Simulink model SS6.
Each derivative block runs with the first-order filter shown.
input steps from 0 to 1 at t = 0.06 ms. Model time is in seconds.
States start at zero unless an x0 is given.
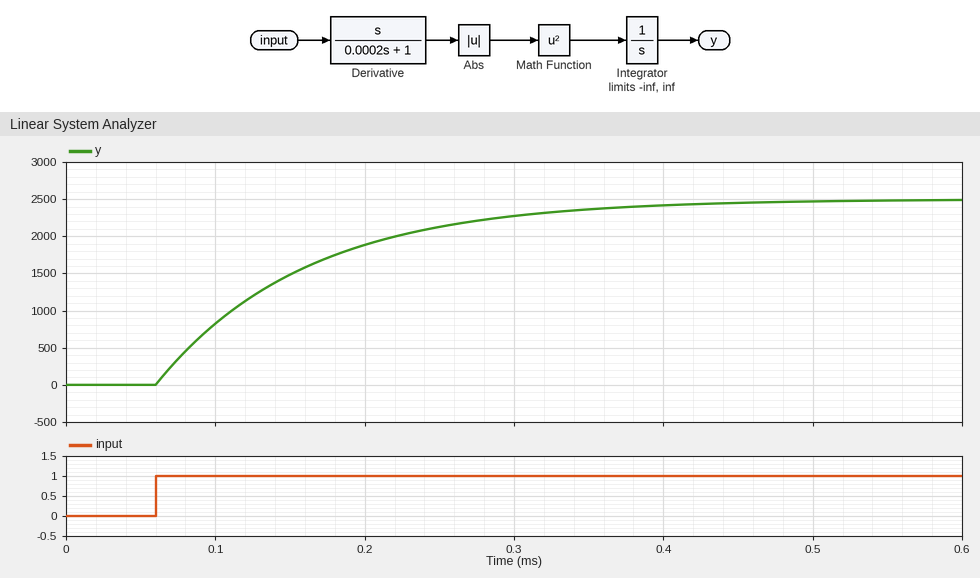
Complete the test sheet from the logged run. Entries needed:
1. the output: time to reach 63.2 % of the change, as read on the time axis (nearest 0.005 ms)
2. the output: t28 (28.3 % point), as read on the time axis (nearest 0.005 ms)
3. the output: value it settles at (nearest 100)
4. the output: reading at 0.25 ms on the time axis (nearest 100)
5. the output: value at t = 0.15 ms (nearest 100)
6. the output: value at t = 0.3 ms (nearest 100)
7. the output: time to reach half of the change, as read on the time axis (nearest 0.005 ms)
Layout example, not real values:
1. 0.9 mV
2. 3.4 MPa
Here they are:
1. 0.160 ms
2. 0.095 ms
3. 2500
4. 2100
5. 1500
6. 2300
7. 0.130 ms
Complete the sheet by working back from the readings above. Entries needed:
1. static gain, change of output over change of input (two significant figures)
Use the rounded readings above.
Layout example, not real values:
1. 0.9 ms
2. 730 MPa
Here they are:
1. 2500
